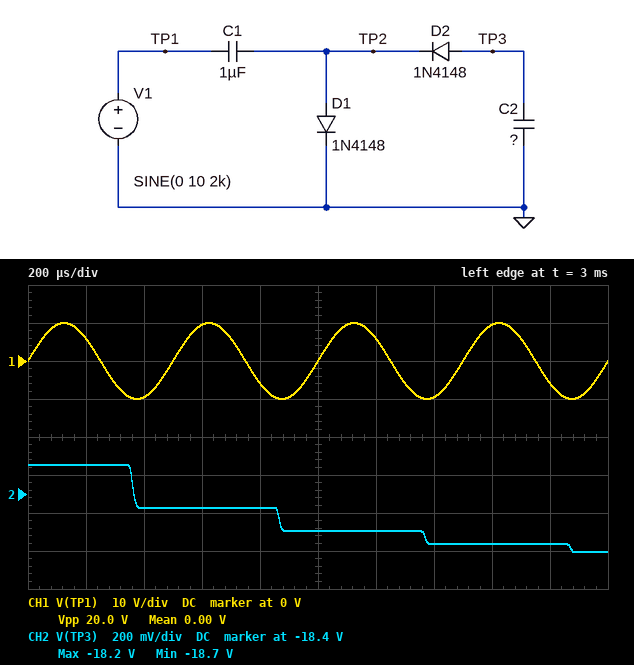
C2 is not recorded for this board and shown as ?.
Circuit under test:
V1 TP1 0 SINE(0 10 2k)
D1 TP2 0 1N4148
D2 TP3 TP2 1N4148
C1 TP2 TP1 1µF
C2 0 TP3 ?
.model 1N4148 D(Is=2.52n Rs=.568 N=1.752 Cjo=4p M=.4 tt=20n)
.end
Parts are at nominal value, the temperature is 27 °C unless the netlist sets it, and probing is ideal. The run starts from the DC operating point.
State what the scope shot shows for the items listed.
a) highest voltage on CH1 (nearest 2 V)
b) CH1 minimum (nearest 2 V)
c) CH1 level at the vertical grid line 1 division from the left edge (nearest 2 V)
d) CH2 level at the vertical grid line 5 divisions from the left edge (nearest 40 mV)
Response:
10 V
-10 V
6 V
-18.60 V
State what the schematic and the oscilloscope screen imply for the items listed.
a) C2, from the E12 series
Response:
1.2 µF
